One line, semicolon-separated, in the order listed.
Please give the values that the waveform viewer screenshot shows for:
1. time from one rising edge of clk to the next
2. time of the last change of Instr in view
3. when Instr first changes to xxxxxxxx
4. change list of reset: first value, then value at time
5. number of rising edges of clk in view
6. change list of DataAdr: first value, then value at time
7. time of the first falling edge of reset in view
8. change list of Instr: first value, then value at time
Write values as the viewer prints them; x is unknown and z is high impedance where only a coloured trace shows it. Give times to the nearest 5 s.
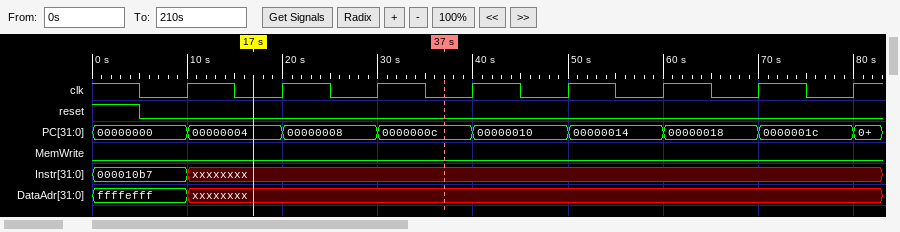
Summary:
10 s; 10 s; 10 s; 1, 0 at 5 s; 8; ffffefff, xxxxxxxx at 10 s; 5 s; 000010b7, xxxxxxxx at 10 s
